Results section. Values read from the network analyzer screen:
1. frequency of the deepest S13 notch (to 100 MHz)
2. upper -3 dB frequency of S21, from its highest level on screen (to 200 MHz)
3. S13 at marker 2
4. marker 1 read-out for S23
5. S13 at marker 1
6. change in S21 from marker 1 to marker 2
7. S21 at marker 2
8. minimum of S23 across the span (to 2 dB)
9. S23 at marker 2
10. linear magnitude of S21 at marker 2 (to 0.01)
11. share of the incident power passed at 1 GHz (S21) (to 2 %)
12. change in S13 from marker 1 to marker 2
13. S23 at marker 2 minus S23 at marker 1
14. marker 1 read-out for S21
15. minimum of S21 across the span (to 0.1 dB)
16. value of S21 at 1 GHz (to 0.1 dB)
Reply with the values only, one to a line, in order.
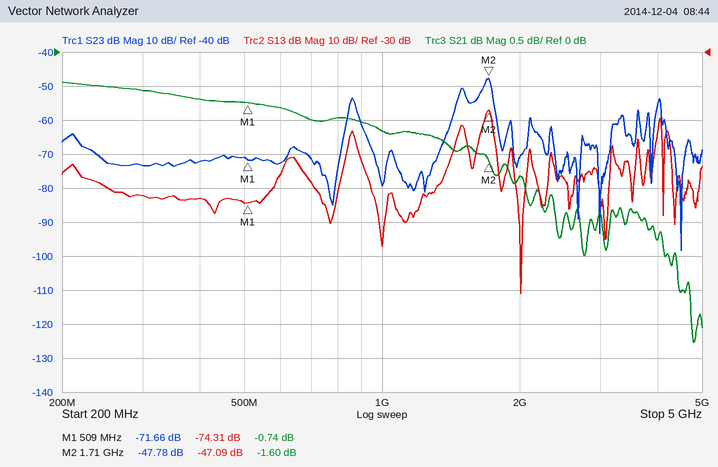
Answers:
2.0 GHz
4.4 GHz
-47.09 dB
-71.66 dB
-74.31 dB
-0.86 dB
-1.60 dB
-98 dB
-47.78 dB
0.83
76 %
27.22 dB
23.88 dB
-0.74 dB
-4.3 dB
-1.2 dB
